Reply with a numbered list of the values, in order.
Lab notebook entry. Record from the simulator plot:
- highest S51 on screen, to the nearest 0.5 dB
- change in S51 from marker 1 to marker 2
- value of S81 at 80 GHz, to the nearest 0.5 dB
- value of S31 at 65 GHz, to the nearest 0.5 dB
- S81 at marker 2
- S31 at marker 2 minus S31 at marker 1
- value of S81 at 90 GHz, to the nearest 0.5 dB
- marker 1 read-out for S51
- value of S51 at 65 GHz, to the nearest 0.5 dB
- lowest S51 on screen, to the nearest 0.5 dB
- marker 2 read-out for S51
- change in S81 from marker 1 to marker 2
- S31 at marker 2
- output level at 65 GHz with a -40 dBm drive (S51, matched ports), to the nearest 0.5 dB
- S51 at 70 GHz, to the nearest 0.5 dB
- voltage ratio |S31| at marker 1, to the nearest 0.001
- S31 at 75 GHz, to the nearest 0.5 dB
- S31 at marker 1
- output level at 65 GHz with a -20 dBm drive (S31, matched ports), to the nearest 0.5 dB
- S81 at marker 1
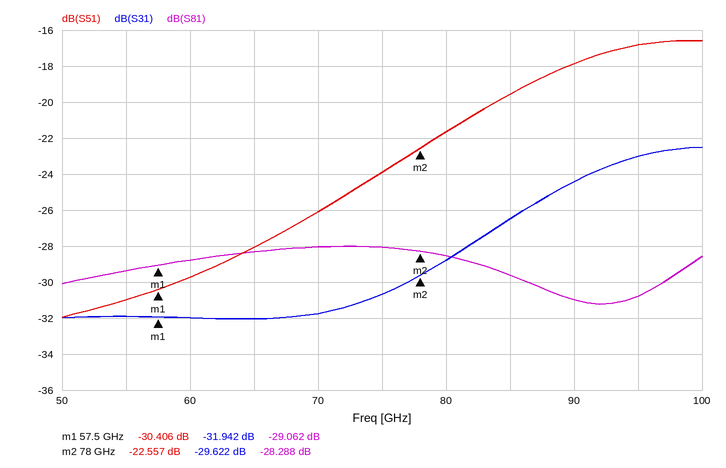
1. -16.5 dB
2. 7.849 dB
3. -28.5 dB
4. -32.0 dB
5. -28.288 dB
6. 2.320 dB
7. -31.0 dB
8. -30.406 dB
9. -28.0 dB
10. -32.0 dB
11. -22.557 dB
12. 0.774 dB
13. -29.622 dB
14. -68.0 dBm
15. -26.0 dB
16. 0.025
17. -30.5 dB
18. -31.942 dB
19. -52.0 dBm
20. -29.062 dB
